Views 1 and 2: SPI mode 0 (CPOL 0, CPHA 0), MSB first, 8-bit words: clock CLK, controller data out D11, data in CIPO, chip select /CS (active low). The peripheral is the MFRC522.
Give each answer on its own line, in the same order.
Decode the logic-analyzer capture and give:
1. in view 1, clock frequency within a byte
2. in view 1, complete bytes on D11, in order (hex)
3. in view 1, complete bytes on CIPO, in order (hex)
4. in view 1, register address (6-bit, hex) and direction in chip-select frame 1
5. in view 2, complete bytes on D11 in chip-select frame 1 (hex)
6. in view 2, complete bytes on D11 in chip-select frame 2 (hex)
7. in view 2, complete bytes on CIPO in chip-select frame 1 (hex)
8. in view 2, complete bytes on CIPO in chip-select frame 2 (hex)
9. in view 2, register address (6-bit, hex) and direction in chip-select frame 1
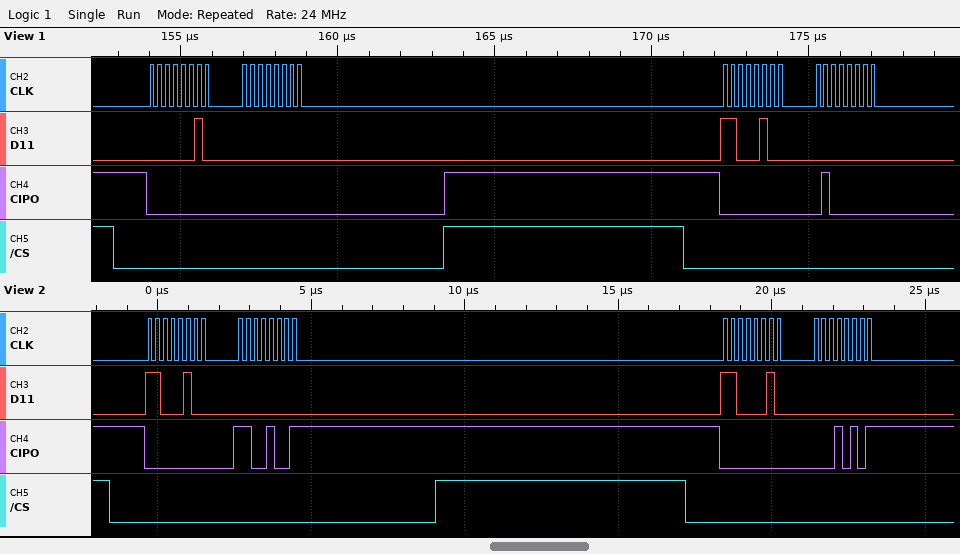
4 MHz
02 00 C4 00
00 00 00 40
0x01 write
C4 00
C2 00
00 C9
00 15
0x22 read
